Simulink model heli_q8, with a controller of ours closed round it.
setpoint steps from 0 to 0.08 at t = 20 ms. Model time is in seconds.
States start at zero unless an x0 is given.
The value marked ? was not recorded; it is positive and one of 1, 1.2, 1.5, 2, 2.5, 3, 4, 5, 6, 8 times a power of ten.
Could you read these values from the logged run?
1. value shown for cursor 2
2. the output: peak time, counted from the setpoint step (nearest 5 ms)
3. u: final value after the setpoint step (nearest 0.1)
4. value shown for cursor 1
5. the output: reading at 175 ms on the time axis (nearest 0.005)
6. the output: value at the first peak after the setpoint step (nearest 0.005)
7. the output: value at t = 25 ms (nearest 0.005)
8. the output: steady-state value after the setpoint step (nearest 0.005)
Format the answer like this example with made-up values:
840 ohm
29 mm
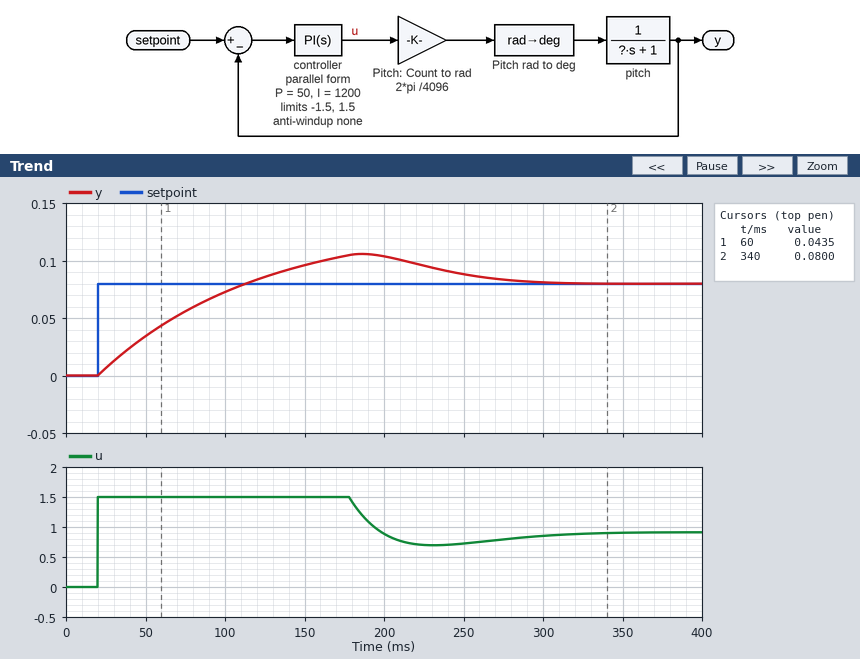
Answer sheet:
0.0800
165 ms
0.9
0.0435
0.105
0.105
0.005
0.080
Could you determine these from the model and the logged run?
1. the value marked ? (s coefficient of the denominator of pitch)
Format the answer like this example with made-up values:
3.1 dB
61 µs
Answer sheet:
0.1
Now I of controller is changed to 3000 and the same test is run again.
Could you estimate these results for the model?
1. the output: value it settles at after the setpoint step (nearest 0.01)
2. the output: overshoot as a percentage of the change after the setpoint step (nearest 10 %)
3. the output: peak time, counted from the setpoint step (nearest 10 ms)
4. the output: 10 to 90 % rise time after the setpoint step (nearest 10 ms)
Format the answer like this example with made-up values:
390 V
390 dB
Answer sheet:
0.08
40 %
200 ms
70 ms
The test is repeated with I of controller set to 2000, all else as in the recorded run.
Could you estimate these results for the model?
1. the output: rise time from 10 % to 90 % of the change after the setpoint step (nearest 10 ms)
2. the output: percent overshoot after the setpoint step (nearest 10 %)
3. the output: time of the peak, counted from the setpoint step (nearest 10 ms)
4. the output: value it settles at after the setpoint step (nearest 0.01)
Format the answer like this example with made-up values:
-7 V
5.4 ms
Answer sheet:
70 ms
40 %
190 ms
0.08
